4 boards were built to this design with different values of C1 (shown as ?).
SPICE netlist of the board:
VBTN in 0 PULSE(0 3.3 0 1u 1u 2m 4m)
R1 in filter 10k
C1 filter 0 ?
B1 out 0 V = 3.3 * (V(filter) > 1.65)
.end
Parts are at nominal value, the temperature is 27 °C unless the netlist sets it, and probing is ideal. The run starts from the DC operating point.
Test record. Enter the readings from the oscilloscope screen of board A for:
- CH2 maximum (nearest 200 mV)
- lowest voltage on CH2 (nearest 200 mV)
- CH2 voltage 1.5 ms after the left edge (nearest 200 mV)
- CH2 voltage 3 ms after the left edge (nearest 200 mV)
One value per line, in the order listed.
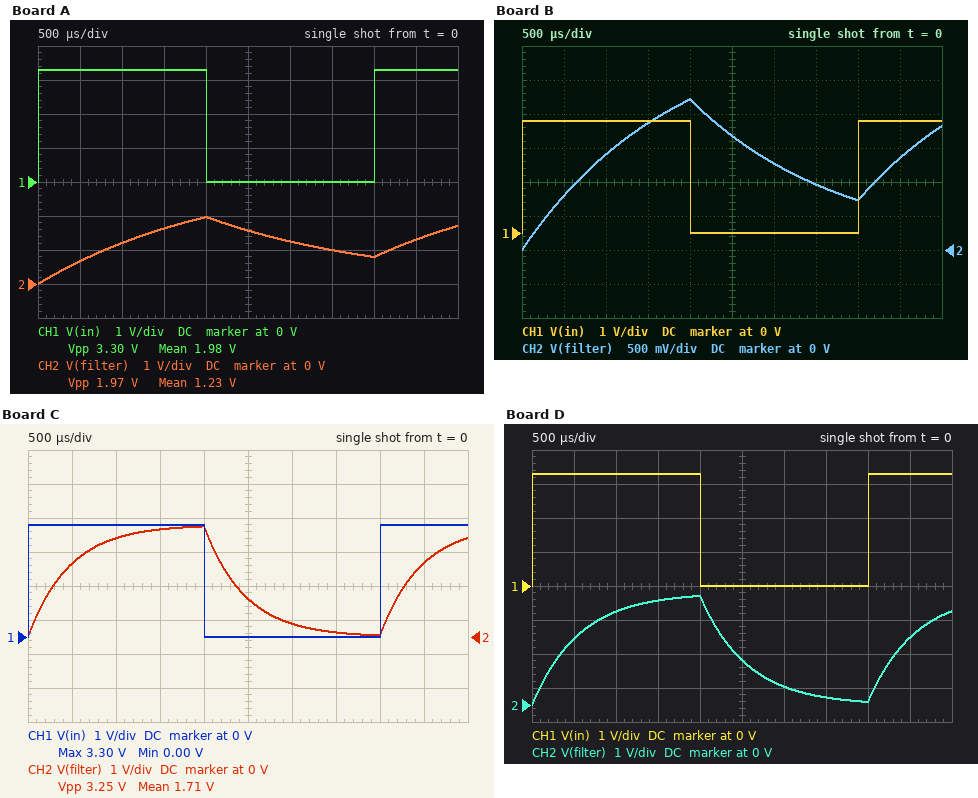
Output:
2.0 V
0 V
1.6 V
1.2 V
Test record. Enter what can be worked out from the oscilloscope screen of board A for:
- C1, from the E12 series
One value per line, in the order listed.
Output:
220 nF
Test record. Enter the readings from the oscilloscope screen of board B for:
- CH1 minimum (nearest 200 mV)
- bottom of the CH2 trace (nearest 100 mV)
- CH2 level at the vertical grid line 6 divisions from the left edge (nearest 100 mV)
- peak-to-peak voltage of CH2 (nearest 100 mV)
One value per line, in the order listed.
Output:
0 V
0 V
1.3 V
2.2 V
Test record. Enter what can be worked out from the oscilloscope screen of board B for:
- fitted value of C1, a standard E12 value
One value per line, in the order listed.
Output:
180 nF
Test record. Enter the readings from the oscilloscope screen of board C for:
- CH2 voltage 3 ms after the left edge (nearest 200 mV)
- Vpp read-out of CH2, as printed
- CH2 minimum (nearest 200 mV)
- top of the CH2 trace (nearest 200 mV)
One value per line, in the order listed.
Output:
400 mV
3.25 V
0 V
3.2 V
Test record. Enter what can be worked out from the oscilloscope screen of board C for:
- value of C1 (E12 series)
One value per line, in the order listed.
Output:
47 nF
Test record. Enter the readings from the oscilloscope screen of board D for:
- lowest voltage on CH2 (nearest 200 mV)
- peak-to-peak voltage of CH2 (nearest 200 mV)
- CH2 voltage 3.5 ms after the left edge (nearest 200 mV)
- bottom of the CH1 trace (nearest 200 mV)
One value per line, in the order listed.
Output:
0 V
3.2 V
200 mV
0 V
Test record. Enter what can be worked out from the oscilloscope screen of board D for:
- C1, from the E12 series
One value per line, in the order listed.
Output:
56 nF
